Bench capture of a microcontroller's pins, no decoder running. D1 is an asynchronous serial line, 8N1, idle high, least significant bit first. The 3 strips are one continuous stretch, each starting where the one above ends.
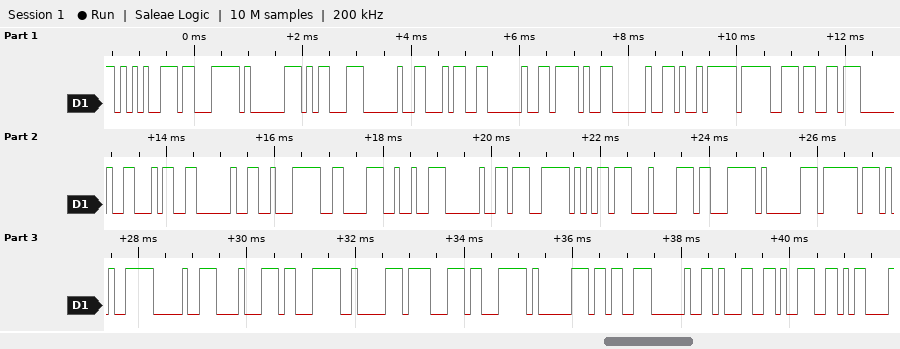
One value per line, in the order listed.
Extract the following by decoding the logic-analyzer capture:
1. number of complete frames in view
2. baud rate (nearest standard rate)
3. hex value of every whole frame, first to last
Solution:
38
9600 baud
95 E3 81 8D 20 34 20 2F 20 E9 9F B3 20 34 20 E2 86 92 20 E7 B5 84 E3 81 BF E5 90 88 E3 82 8F E3 81 9B 20 31 39 0D
